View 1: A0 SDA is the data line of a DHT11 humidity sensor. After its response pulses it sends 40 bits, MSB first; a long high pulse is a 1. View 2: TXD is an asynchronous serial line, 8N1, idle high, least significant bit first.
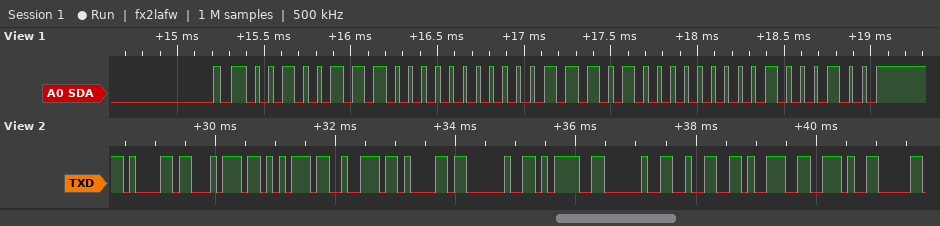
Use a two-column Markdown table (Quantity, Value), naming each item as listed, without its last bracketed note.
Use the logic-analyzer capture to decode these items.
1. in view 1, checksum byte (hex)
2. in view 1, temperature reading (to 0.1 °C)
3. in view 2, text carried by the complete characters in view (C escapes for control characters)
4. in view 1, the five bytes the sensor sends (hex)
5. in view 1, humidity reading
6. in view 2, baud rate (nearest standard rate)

| Quantity | Value |
|---|---|
| in view 1, checksum byte | 0x44 |
| in view 1, temperature reading | 29.0 °C |
| in view 2, text carried by the complete characters in view | "atura = 29." |
| in view 1, the five bytes the sensor sends | 27 00 1D 00 44 |
| in view 1, humidity reading | 39 % |
| in view 2, baud rate | 9600 baud |
